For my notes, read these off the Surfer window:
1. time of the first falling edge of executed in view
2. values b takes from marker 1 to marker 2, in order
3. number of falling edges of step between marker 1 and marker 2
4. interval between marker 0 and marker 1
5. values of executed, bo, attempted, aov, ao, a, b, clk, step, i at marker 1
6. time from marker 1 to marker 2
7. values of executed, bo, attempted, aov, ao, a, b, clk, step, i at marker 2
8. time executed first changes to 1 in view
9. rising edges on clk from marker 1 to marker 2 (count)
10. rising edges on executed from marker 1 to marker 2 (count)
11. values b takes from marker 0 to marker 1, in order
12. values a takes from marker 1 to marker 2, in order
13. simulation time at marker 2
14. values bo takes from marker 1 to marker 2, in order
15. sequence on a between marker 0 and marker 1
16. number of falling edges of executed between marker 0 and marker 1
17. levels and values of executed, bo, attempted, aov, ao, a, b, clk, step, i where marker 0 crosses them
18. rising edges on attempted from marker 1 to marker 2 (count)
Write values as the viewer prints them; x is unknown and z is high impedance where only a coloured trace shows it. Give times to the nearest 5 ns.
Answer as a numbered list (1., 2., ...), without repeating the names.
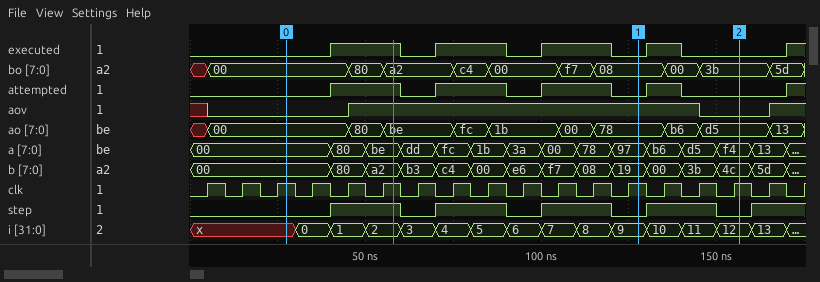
1. 60 ns
2. 19, 00, 3b, 4c
3. 1
4. 100 ns
5. executed=0, bo=08, attempted=0, aov=1, ao=78, a=97, b=19, clk=1, step=0, i=9
6. 30 ns
7. executed=0, bo=3b, attempted=0, aov=0, ao=d5, a=f4, b=4c, clk=1, step=0, i=12
8. 40 ns
9. 3
10. 1
11. 00, 80, a2, b3, c4, 00, e6, f7, 08, 19
12. 97, b6, d5, f4
13. 155 ns
14. 08, 00, 3b
15. 00, 80, be, dd, fc, 1b, 3a, 00, 78, 97
16. 3
17. executed=0, bo=00, attempted=0, aov=0, ao=00, a=00, b=00, clk=1, step=0, i=x
18. 1
